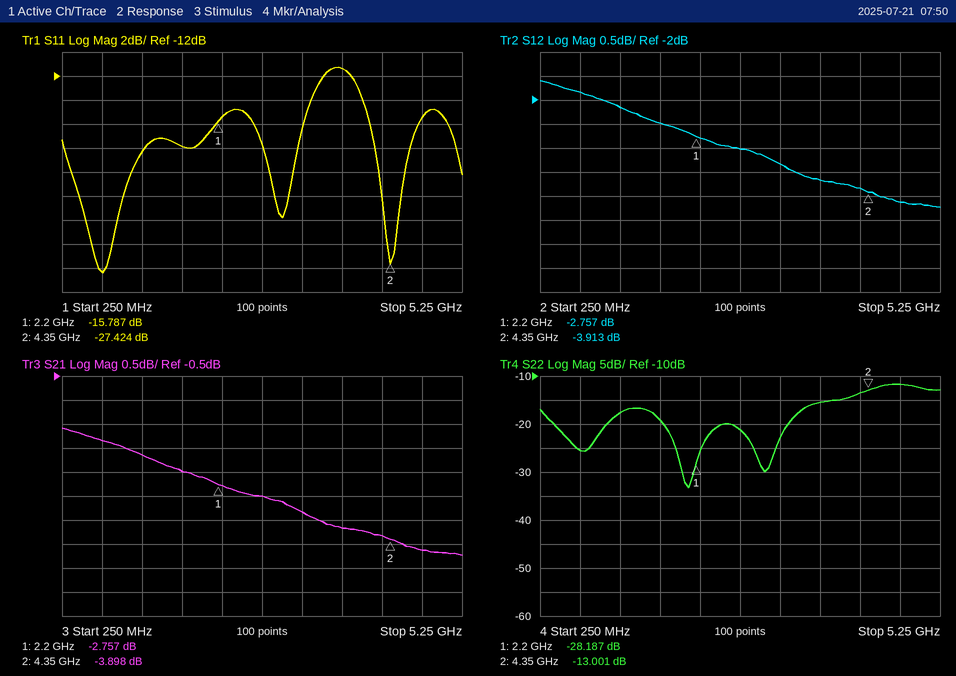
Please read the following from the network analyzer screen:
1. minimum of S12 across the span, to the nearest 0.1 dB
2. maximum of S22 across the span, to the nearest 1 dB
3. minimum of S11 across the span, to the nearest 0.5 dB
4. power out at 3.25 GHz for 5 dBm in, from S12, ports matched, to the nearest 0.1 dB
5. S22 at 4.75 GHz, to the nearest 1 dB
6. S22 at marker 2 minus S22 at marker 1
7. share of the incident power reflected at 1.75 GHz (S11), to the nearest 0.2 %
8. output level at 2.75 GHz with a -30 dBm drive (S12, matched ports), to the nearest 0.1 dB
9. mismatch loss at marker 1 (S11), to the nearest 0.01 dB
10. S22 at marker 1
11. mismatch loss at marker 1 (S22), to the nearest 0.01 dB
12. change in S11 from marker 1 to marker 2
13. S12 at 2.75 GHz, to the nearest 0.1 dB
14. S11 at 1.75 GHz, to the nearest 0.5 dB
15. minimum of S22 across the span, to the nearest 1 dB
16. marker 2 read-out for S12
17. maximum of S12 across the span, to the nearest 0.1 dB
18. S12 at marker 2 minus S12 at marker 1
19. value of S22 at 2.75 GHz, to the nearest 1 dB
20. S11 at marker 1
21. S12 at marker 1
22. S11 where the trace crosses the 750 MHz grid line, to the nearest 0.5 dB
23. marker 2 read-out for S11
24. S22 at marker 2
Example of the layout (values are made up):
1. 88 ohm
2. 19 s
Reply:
1. -4.2 dB
2. -12 dB
3. -28.5 dB
4. 1.7 dBm
5. -12 dB
6. 15.186 dB
7. 1.6 %
8. -33.0 dBm
9. 0.12 dB
10. -28.187 dB
11. 0.01 dB
12. -11.637 dB
13. -3.0 dB
14. -18.0 dB
15. -33 dB
16. -3.913 dB
17. -1.6 dB
18. -1.156 dB
19. -21 dB
20. -15.787 dB
21. -2.757 dB
22. -28.5 dB
23. -27.424 dB
24. -13.001 dB
